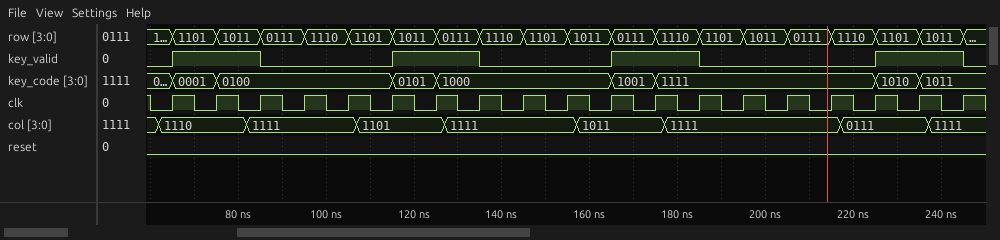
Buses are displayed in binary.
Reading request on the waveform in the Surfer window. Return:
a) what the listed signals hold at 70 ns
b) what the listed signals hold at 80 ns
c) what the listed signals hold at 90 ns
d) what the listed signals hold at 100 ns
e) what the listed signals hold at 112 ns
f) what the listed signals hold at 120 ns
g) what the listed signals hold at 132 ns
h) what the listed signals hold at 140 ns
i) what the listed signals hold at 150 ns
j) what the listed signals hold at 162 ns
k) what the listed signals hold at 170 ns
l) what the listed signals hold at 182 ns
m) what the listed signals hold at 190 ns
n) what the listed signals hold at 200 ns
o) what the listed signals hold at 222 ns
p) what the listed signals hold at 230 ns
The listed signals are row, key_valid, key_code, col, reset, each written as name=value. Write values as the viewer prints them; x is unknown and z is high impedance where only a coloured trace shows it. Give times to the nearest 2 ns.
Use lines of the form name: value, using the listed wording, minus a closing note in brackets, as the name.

what the listed signals hold at 70 ns: row=1101, key_valid=1, key_code=0001, col=1110, reset=0
what the listed signals hold at 80 ns: row=1011, key_valid=1, key_code=0100, col=1110, reset=0
what the listed signals hold at 90 ns: row=0111, key_valid=0, key_code=0100, col=1111, reset=0
what the listed signals hold at 100 ns: row=1110, key_valid=0, key_code=0100, col=1111, reset=0
what the listed signals hold at 112 ns: row=1101, key_valid=0, key_code=0100, col=1101, reset=0
what the listed signals hold at 120 ns: row=1011, key_valid=1, key_code=0101, col=1101, reset=0
what the listed signals hold at 132 ns: row=0111, key_valid=1, key_code=1000, col=1111, reset=0
what the listed signals hold at 140 ns: row=1110, key_valid=0, key_code=1000, col=1111, reset=0
what the listed signals hold at 150 ns: row=1101, key_valid=0, key_code=1000, col=1111, reset=0
what the listed signals hold at 162 ns: row=1011, key_valid=0, key_code=1000, col=1011, reset=0
what the listed signals hold at 170 ns: row=0111, key_valid=1, key_code=1001, col=1011, reset=0
what the listed signals hold at 182 ns: row=1110, key_valid=1, key_code=1111, col=1111, reset=0
what the listed signals hold at 190 ns: row=1101, key_valid=0, key_code=1111, col=1111, reset=0
what the listed signals hold at 200 ns: row=1011, key_valid=0, key_code=1111, col=1111, reset=0
what the listed signals hold at 222 ns: row=1110, key_valid=0, key_code=1111, col=0111, reset=0
what the listed signals hold at 230 ns: row=1101, key_valid=1, key_code=1010, col=0111, reset=0
